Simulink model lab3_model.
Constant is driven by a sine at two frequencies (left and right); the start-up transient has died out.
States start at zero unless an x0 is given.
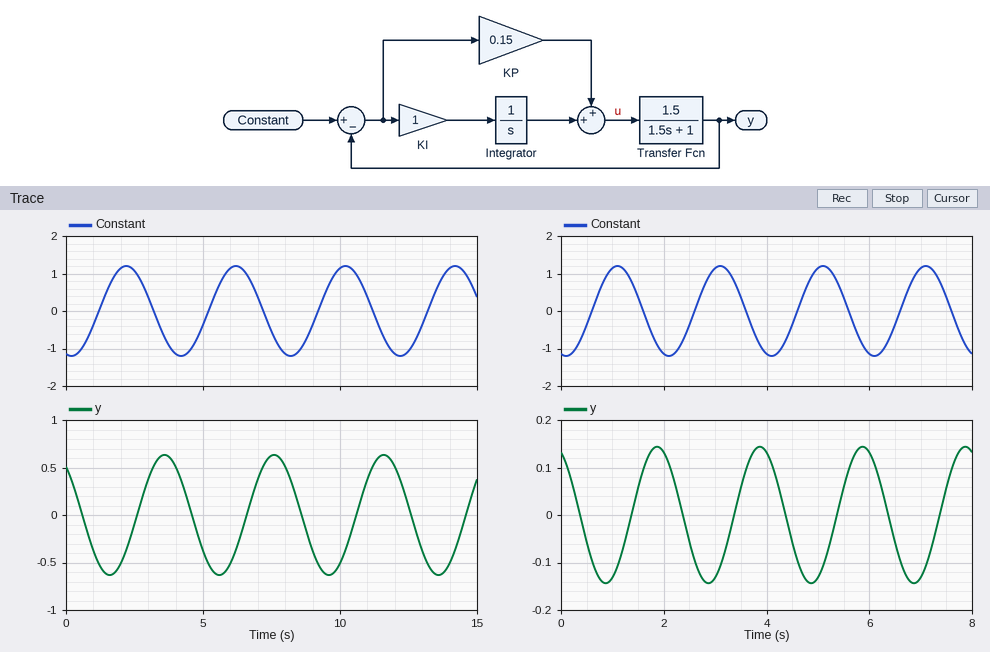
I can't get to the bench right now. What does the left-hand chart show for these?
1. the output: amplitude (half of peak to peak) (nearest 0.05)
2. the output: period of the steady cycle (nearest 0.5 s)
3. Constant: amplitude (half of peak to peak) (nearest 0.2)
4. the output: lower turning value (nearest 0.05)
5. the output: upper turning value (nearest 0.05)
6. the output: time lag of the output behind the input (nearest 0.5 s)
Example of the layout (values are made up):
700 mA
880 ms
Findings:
0.65
4.0 s
1.2
-0.65
0.65
1.5 s
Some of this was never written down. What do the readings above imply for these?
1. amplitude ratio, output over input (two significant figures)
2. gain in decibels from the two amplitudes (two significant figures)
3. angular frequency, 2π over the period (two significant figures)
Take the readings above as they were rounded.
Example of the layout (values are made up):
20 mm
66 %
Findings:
0.54
-5.3 dB
1.6 rad/s
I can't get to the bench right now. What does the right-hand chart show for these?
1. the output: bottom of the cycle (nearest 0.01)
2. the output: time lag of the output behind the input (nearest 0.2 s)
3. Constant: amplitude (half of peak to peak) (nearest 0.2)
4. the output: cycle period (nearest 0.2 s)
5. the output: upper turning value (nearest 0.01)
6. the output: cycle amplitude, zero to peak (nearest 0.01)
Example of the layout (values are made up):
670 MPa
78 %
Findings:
-0.14
0.8 s
1.2
2.0 s
0.14
0.14
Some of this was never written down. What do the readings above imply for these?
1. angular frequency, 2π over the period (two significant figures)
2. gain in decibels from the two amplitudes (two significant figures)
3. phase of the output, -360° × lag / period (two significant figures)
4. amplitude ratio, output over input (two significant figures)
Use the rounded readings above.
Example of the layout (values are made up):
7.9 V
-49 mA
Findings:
3.1 rad/s
-19 dB
-140°
0.12
